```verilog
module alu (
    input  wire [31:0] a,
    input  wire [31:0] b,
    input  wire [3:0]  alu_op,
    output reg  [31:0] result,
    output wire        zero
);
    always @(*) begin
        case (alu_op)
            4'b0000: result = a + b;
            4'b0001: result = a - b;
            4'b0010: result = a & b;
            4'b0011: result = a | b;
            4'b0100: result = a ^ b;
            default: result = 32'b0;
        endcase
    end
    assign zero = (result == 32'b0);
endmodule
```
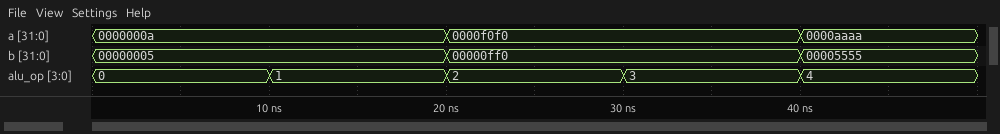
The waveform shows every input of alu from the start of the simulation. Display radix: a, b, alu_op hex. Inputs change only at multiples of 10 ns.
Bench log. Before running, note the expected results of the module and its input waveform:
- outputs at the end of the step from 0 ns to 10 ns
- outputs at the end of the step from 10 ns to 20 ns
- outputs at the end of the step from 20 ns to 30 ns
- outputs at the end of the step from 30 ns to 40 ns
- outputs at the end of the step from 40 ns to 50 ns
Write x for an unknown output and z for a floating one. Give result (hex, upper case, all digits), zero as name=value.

result=0000000F, zero=0
result=00000005, zero=0
result=000000F0, zero=0
result=0000FFF0, zero=0
result=0000FFFF, zero=0
